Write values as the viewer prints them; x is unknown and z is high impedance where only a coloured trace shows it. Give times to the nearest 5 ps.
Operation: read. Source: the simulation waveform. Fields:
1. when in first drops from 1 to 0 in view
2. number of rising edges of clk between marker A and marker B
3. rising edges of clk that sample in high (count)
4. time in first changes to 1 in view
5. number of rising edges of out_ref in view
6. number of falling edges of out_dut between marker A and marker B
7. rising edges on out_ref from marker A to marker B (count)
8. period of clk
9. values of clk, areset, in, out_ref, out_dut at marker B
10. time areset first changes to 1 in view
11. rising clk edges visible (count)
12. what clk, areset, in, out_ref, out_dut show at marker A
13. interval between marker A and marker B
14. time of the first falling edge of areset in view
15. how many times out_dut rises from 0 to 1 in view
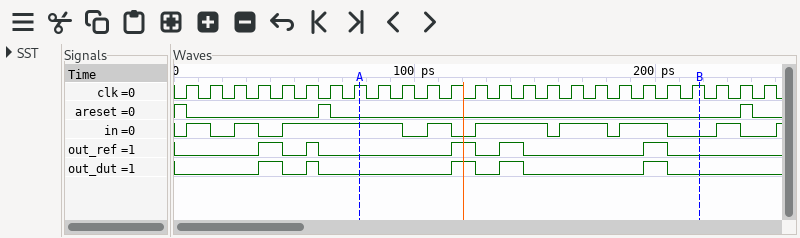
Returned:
15 ps
14
16
5 ps
5
3
3
10 ps
clk=1, areset=0, in=0, out_ref=0, out_dut=0
60 ps
25
clk=1, areset=0, in=1, out_ref=0, out_dut=0
140 ps
5 ps
5
